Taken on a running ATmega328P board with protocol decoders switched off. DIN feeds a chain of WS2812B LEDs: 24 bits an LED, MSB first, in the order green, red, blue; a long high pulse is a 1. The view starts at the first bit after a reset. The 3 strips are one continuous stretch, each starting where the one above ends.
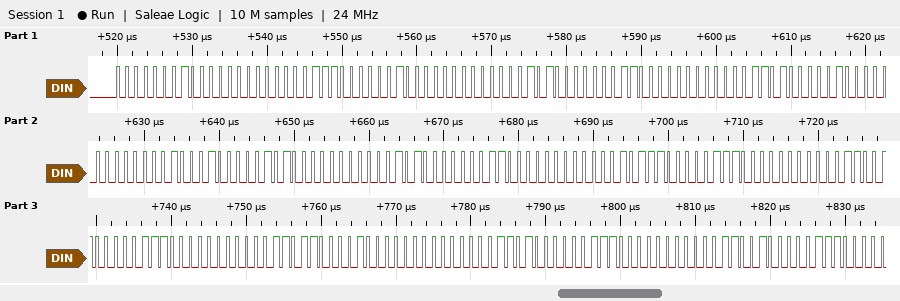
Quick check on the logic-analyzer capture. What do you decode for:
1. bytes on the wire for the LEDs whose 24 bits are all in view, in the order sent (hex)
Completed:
01 00 07 02 00 0A 03 00 0D 04 00 11 05 00 14 06 00 17 07 00 19 07 00 1B 08 00 1A 07 00 19
